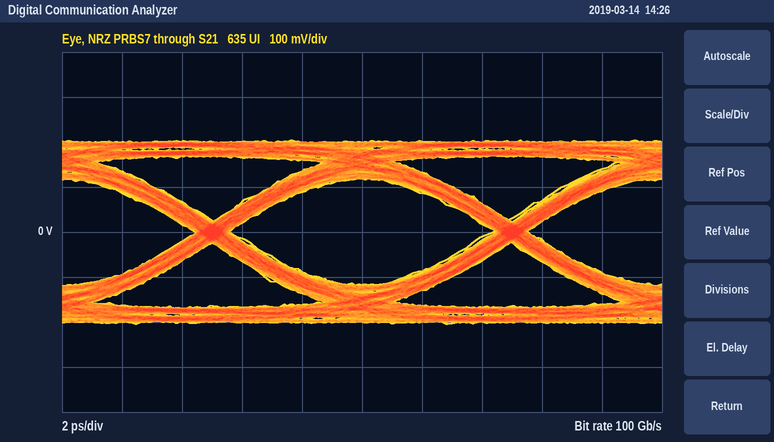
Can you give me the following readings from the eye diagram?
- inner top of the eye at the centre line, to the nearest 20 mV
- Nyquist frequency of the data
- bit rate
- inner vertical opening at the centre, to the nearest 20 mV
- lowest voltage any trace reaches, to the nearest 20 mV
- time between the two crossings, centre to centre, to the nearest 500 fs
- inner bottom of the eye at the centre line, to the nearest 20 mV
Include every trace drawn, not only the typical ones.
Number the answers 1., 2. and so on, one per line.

1. 120 mV
2. 50 GHz
3. 100 Gb/s
4. 240 mV
5. -200 mV
6. 10.0 ps
7. -120 mV
